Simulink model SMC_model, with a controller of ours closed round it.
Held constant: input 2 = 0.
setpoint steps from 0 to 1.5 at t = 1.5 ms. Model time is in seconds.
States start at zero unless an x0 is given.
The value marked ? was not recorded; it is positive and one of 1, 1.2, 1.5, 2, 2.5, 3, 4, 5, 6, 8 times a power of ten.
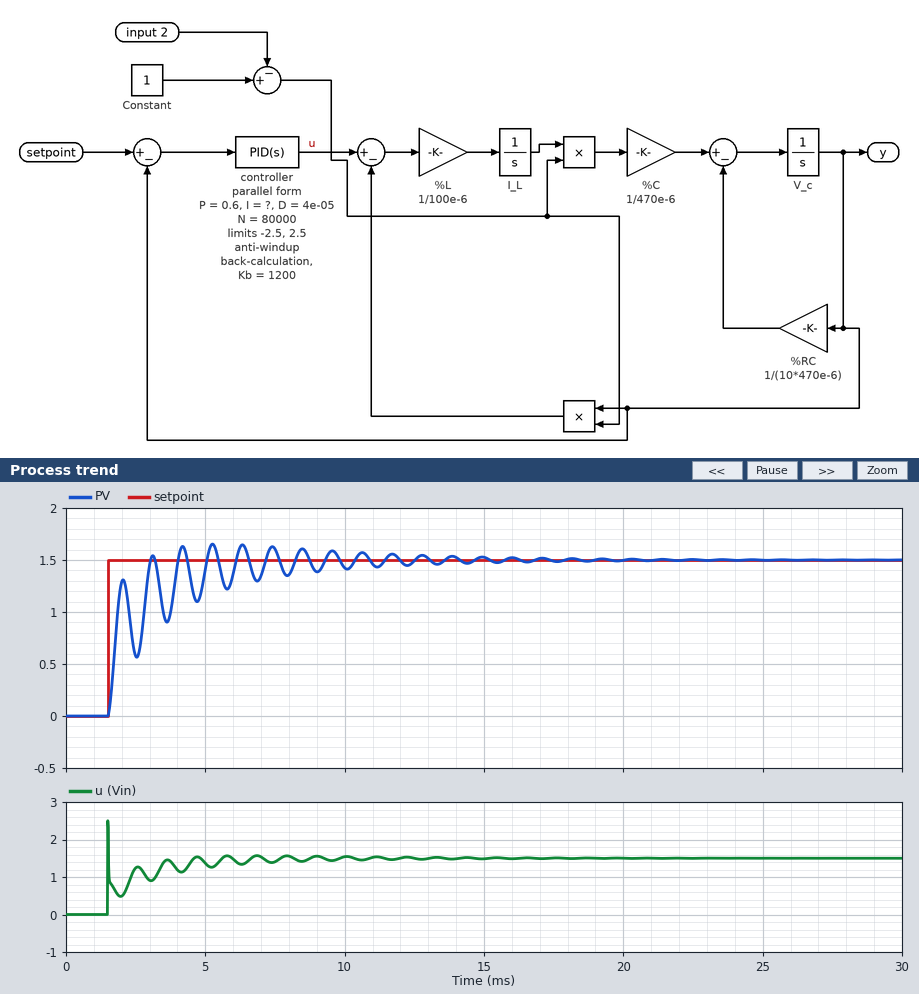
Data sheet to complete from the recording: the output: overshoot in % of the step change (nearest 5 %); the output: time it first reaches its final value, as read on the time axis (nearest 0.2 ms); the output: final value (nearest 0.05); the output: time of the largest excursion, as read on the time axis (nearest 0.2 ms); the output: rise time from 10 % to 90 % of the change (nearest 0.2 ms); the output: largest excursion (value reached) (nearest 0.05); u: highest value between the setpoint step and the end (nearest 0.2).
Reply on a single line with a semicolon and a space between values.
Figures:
10 %; 3.0 ms; 1.50; 5.2 ms; 1.4 ms; 1.65; 2.4
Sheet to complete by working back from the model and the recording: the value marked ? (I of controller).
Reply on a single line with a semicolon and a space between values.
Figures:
1000
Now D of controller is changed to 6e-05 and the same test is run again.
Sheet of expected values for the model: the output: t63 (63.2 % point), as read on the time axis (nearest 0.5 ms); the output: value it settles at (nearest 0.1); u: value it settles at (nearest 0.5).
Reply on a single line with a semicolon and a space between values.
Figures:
2.0 ms; 1.5; 1.5
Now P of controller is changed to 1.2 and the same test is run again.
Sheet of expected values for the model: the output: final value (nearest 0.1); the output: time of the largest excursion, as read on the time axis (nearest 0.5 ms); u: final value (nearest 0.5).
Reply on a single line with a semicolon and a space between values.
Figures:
1.5; 3.0 ms; 1.5
